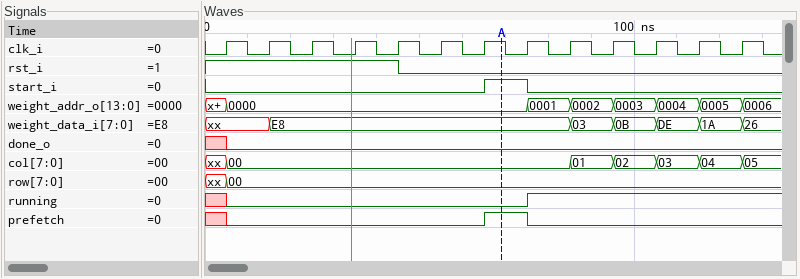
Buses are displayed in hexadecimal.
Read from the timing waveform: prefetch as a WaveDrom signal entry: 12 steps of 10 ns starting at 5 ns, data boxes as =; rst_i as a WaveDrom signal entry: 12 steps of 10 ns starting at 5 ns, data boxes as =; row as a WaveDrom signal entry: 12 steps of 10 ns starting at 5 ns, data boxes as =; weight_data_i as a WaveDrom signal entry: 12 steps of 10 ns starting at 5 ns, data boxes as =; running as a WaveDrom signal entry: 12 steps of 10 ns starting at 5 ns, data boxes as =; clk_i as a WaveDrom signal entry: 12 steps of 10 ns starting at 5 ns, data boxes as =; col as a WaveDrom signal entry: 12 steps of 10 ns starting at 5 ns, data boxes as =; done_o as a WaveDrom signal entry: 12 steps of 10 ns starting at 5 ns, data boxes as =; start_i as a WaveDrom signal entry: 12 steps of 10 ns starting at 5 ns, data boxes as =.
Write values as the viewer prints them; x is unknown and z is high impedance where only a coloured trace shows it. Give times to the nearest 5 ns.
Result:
{name: 'prefetch', wave: '0.....10....'}
{name: 'rst_i', wave: '1...0.......'}
{name: 'row', wave: '=...........', data: '00'}
{name: 'weight_data_i', wave: 'x=......====', data: 'E8 03 0B DE 1A'}
{name: 'running', wave: '0......1....'}
{name: 'clk_i', wave: 'p...........'}
{name: 'col', wave: '=.......====', data: '00 01 02 03 04'}
{name: 'done_o', wave: '0...........'}
{name: 'start_i', wave: '0.....10....'}
